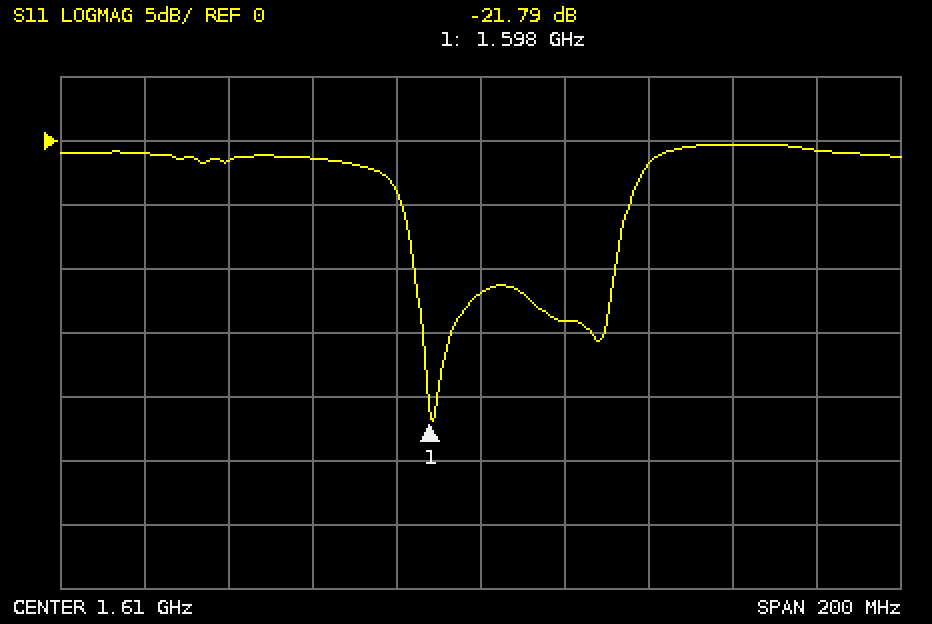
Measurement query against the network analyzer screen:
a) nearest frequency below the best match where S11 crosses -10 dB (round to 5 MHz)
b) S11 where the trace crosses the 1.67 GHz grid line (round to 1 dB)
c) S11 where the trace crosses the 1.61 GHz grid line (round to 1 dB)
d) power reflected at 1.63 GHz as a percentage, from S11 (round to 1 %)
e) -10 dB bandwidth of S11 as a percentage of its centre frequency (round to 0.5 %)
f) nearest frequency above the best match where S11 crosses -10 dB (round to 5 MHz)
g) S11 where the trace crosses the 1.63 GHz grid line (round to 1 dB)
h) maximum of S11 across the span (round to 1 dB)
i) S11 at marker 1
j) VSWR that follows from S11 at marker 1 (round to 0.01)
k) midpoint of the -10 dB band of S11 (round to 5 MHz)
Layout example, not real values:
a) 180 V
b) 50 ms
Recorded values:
a) 1.595 GHz
b) 0 dB
c) -12 dB
d) 4 %
e) 3.0 %
f) 1.640 GHz
g) -14 dB
h) 0 dB
i) -21.79 dB
j) 1.18
k) 1.620 GHz
